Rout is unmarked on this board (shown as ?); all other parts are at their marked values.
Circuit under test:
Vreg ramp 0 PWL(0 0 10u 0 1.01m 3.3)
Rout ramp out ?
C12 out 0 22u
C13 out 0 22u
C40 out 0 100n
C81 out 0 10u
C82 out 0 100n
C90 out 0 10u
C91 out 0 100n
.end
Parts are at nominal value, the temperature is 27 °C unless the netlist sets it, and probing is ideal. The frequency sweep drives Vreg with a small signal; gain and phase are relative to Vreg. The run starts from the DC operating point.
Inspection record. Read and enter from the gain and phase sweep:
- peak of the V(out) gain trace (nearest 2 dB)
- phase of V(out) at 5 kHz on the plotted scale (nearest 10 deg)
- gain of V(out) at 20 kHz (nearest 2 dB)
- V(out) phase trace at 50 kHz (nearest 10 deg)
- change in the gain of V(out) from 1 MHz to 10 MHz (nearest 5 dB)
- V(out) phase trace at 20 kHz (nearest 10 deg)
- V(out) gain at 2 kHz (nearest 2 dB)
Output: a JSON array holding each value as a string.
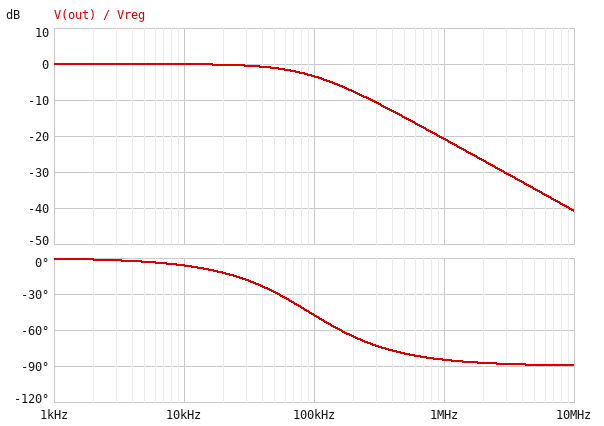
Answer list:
["0 dB", "0 deg", "0 dB", "-30 deg", "-20 dB", "-10 deg", "0 dB"]
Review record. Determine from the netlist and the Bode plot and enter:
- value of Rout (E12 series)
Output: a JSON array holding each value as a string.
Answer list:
["0.027 Ω"]
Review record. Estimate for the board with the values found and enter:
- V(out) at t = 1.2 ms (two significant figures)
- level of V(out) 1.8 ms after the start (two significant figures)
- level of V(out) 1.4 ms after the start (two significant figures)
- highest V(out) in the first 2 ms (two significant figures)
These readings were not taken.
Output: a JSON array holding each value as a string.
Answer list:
["3.3 V", "3.3 V", "3.3 V", "3.3 V"]
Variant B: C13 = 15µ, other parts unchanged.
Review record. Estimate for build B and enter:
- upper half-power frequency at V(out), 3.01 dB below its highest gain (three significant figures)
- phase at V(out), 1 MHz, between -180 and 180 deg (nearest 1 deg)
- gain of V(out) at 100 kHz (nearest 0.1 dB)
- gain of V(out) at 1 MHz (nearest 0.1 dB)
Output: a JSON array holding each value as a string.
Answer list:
["103 kHz", "-84 deg", "-2.9 dB", "-19.8 dB"]
